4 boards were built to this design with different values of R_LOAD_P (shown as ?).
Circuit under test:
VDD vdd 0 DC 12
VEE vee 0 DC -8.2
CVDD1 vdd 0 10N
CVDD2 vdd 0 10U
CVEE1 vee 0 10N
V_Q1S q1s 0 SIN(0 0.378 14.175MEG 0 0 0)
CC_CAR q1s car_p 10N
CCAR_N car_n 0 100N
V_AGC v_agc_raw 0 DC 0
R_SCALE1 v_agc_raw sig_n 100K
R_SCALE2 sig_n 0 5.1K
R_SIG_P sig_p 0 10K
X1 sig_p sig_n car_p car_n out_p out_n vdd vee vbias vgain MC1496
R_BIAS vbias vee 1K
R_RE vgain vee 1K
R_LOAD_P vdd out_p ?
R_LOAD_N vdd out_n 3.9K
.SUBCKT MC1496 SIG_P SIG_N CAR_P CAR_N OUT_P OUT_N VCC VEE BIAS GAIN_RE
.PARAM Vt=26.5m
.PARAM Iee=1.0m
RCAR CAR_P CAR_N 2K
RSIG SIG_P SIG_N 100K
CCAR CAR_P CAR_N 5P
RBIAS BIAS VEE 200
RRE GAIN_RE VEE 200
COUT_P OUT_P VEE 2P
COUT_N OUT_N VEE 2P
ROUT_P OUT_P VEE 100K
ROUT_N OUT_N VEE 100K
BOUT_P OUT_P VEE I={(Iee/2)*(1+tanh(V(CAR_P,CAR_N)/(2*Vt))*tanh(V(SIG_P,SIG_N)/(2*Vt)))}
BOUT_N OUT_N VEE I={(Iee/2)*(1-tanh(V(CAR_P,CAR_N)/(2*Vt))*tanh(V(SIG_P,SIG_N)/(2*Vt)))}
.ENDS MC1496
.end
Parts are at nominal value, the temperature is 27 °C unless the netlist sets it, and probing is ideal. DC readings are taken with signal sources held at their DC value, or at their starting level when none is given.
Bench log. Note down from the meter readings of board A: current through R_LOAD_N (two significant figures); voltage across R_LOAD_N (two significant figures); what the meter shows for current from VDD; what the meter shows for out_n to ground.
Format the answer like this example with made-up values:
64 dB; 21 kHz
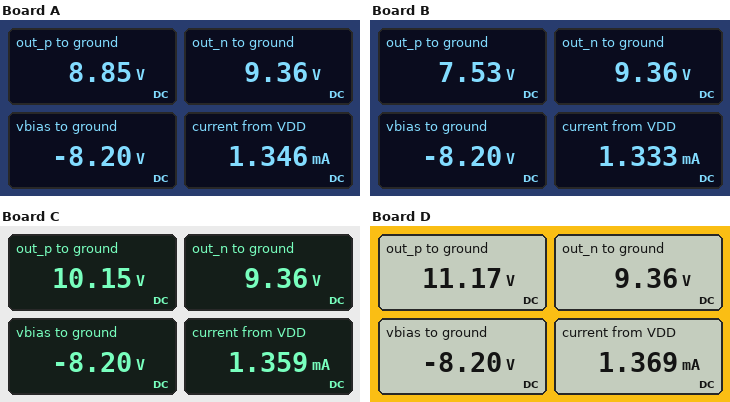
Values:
680 µA; 2.6 V; 1.346 mA; 9.36 V
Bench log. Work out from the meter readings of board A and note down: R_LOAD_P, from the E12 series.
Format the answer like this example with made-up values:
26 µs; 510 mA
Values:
4.7 kΩ
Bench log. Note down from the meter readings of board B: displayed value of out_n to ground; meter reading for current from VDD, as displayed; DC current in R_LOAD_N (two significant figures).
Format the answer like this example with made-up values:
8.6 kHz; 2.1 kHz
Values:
9.36 V; 1.333 mA; 680 µA
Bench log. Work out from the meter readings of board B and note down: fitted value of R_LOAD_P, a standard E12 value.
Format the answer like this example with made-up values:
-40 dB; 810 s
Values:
6.8 kΩ
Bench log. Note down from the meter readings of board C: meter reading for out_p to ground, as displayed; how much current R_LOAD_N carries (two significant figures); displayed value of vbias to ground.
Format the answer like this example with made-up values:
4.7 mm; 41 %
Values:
10.15 V; 680 µA; -8.20 V
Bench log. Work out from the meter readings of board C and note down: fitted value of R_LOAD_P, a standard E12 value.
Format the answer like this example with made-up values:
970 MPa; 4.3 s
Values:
2.7 kΩ
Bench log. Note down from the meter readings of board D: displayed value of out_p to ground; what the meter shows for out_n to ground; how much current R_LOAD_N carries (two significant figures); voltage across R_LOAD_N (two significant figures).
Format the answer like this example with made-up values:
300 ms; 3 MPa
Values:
11.17 V; 9.36 V; 680 µA; 2.6 V
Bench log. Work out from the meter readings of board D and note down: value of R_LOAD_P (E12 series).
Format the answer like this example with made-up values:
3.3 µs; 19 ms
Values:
1.2 kΩ
